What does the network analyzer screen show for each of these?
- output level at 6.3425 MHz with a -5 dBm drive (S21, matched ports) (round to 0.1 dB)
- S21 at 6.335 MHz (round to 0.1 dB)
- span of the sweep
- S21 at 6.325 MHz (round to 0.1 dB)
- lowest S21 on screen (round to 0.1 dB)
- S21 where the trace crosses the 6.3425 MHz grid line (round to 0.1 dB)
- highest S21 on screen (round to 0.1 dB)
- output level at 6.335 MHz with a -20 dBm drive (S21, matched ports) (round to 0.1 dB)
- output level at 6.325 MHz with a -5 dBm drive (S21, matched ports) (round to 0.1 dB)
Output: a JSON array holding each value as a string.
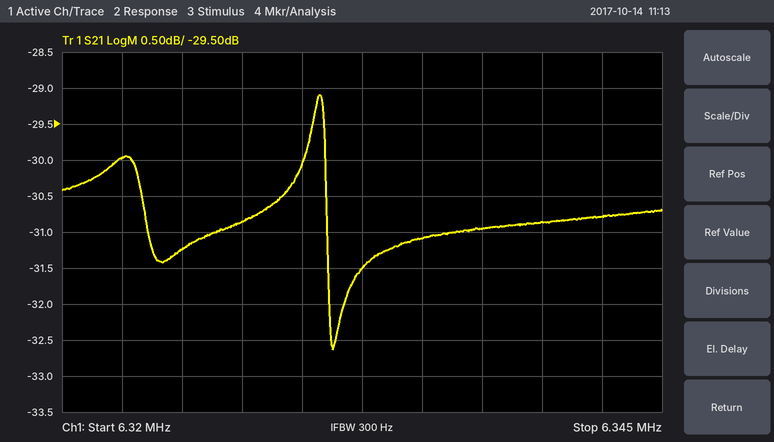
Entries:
["-35.8 dBm", "-31.1 dB", "25 kHz", "-31.2 dB", "-32.6 dB", "-30.8 dB", "-29.1 dB", "-51.1 dBm", "-36.2 dBm"]
